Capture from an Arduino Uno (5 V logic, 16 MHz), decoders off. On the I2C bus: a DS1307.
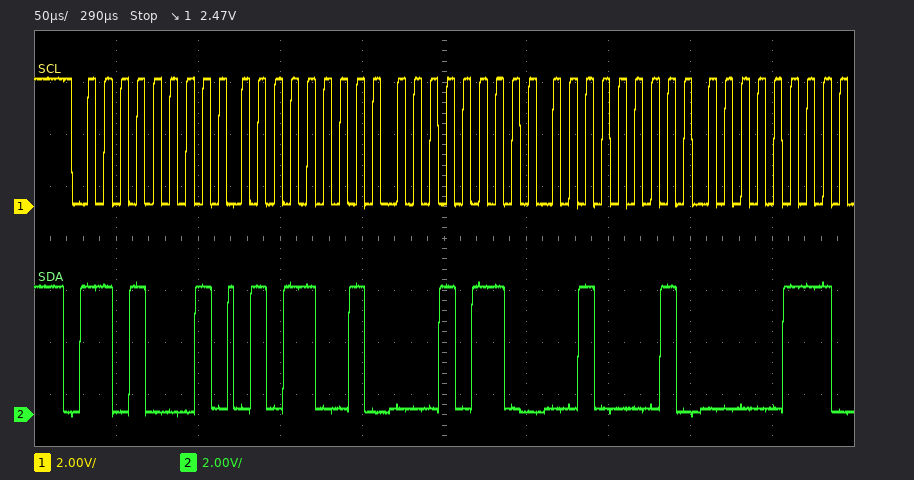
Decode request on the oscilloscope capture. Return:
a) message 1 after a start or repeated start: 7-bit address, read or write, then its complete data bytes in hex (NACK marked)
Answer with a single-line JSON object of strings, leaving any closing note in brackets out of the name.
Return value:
{"message 1 after a start or repeated start: 7-bit address, read or write, then its complete data bytes in hex": "0x68 read: 59 16 21 07"}
